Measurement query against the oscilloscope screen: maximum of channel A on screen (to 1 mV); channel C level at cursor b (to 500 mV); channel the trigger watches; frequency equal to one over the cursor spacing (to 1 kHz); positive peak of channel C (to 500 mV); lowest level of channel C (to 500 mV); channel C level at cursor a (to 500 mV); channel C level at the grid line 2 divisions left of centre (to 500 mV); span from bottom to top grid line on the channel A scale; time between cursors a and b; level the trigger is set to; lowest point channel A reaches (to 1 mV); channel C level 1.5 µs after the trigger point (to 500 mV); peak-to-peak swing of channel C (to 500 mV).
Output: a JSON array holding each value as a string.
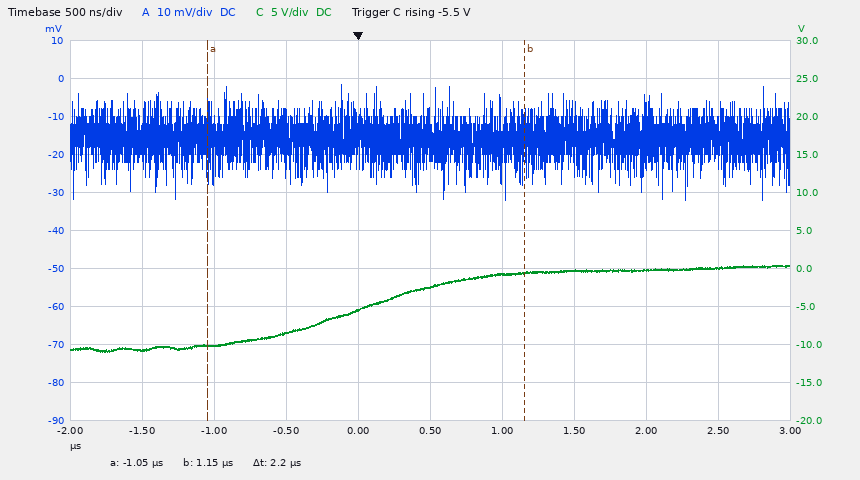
["-2 mV", "-500 mV", "channel C", "455 kHz", "500 mV", "-11.0 V", "-10.0 V", "-8.5 V", "100 mV", "2.2 µs", "-5.5 V", "-32 mV", "-500 mV", "11.5 V"]
